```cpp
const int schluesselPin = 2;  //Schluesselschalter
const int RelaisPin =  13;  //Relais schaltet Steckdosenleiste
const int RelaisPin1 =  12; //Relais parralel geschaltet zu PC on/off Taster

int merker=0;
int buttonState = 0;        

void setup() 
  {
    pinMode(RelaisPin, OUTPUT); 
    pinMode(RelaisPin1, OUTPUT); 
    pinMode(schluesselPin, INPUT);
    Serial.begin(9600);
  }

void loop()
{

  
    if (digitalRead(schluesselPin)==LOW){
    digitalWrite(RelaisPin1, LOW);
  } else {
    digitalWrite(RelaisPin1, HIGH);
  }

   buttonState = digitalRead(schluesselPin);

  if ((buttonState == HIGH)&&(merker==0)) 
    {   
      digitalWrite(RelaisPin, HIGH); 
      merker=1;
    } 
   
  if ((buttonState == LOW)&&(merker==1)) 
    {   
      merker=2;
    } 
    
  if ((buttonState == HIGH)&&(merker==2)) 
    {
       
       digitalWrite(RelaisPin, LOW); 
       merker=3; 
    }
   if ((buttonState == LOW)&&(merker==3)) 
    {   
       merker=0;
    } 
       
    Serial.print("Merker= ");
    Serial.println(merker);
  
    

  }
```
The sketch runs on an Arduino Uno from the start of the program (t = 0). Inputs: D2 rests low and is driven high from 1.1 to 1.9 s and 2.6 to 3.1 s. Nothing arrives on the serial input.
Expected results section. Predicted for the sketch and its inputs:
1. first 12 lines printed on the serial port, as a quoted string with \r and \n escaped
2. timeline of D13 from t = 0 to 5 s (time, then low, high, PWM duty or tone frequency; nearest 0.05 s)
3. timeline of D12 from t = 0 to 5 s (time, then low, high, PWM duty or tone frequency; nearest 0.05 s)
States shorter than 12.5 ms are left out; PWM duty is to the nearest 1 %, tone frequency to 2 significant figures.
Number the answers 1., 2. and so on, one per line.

1. "Merker= 0\r\nMerker= 0\r\nMerker= 0\r\nMerker= 0\r\nMerker= 0\r\nMerker= 0\r\nMerker= 0\r\nMerker= 0\r\nMerker= 0\r\nMerker= 0\r\nMerker= 0\r\nMerker= 0\r\n"
2. 0 s low; 1.1 s high; 2.6 s low
3. 0 s low; 1.1 s high; 1.9 s low; 2.6 s high; 3.1 s low
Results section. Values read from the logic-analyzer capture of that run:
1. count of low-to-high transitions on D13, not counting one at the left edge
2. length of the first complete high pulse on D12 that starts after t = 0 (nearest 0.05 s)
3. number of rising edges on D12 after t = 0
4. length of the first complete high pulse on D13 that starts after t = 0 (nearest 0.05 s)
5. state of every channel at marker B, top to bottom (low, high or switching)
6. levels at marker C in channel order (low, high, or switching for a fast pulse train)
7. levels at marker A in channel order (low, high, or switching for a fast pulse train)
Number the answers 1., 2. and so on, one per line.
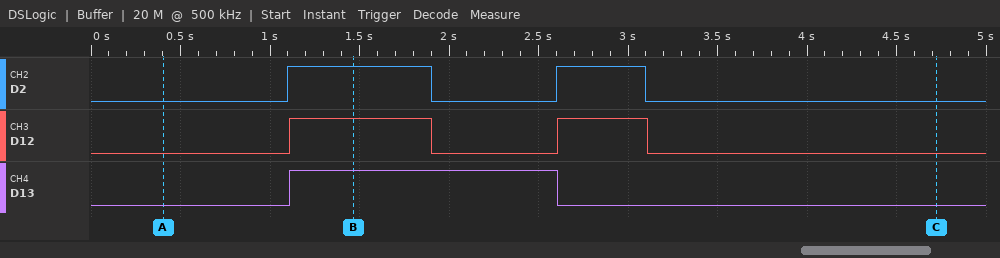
1. 1
2. 0.80 s
3. 2
4. 1.50 s
5. D2 high, D12 high, D13 high
6. D2 low, D12 low, D13 low
7. D2 low, D12 low, D13 low
